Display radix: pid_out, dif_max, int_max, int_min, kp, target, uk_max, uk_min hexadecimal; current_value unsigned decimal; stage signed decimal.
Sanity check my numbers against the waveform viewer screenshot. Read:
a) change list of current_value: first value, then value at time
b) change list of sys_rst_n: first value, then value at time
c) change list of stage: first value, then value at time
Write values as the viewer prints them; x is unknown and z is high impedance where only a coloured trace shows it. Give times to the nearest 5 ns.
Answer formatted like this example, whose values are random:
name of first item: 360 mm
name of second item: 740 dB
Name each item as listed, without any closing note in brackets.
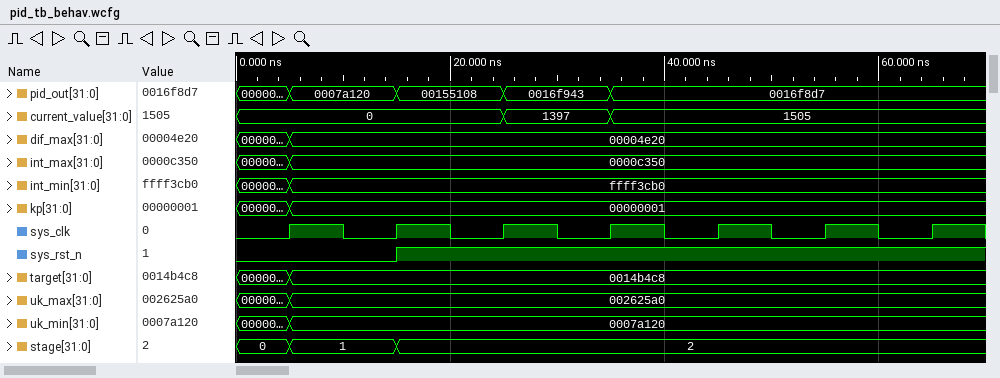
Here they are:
change list of current_value: first value, then value at time: 0, 1397 at 25 ns, 1505 at 35 ns
change list of sys_rst_n: first value, then value at time: 0, 1 at 15 ns
change list of stage: first value, then value at time: 0, 1 at 5 ns, 2 at 15 ns
